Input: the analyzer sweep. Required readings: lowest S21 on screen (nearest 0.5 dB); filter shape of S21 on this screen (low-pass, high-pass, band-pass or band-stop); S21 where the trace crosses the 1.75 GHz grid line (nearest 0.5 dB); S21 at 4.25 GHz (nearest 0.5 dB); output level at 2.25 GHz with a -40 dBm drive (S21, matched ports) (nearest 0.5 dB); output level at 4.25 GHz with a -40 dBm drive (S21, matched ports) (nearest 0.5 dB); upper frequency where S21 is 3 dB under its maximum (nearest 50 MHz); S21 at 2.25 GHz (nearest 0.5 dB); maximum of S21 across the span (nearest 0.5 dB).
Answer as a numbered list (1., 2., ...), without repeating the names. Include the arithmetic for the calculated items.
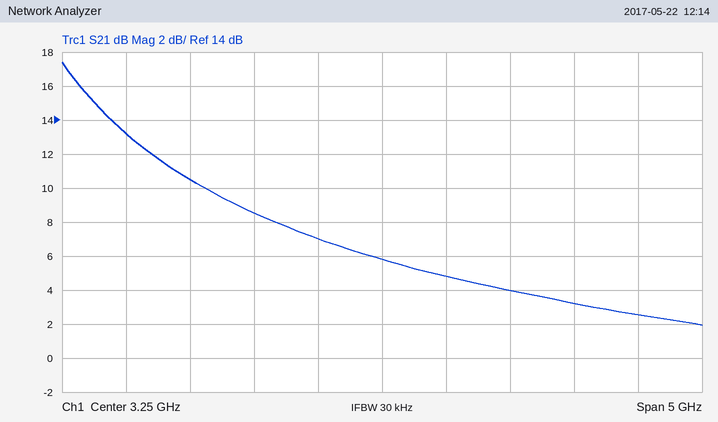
1. 2.0 dB
2. low-pass
3. 10.5 dB
4. 4.0 dB
5. -40 dBm + (8.5 dB) = -31.5 dBm
6. -40 dBm + (4.0 dB) = -36.0 dBm
7. 1.10 GHz
8. 8.5 dB
9. 17.5 dB
